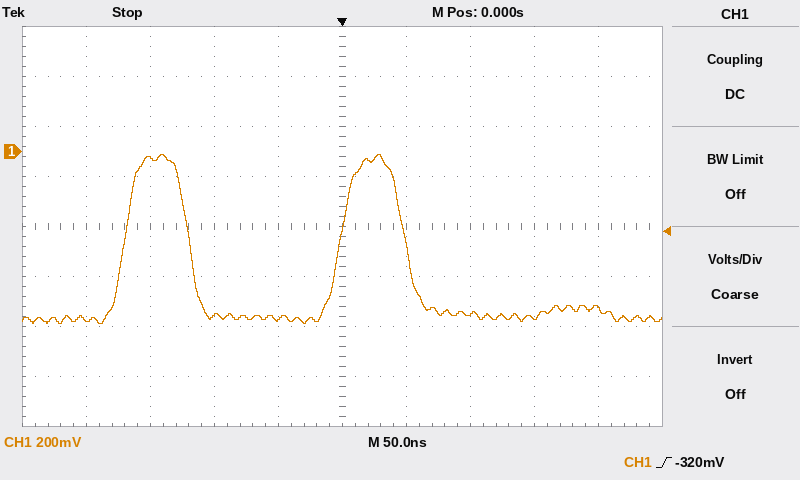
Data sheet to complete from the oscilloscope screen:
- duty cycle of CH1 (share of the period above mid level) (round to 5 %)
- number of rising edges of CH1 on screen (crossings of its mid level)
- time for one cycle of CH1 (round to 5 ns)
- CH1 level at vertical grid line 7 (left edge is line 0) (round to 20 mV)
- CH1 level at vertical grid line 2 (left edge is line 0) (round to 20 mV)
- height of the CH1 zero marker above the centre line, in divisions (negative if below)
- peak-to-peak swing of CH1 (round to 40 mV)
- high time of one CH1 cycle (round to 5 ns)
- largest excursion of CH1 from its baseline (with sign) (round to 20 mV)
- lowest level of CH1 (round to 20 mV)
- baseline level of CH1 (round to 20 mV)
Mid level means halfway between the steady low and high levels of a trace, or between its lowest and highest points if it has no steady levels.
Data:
30 %
2
170 ns
-640 mV
-20 mV
+1.5 div
680 mV
50 ns
+640 mV
-680 mV
-660 mV
